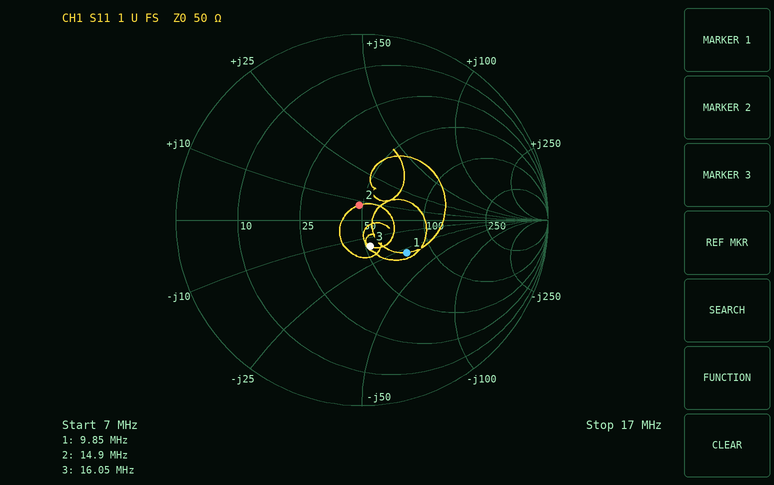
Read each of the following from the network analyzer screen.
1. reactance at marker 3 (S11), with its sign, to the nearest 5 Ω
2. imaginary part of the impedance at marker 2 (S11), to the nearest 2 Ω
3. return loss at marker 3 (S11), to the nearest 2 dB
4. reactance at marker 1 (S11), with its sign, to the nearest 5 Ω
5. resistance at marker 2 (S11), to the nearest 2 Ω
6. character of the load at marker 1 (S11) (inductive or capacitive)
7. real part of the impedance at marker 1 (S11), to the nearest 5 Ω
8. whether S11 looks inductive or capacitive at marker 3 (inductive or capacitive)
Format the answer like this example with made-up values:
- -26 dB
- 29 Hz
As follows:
- -15 Ω
- +8 Ω
- 16 dB
- -30 Ω
- 48 Ω
- capacitive
- 75 Ω
- capacitive
